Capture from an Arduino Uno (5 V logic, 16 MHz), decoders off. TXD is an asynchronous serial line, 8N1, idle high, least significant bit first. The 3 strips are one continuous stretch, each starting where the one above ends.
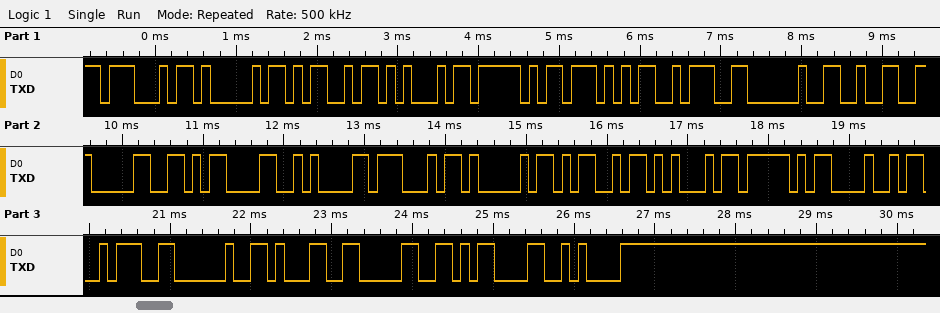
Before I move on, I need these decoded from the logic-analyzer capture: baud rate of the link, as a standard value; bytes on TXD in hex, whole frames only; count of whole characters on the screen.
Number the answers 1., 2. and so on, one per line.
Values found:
1. 9600 baud
2. 47 41 4D 45 5F 57 3A 20 32 30 0D 0A 47 41 4D 45 5F 48 3A 20 31 30 0D 0A
3. 24
